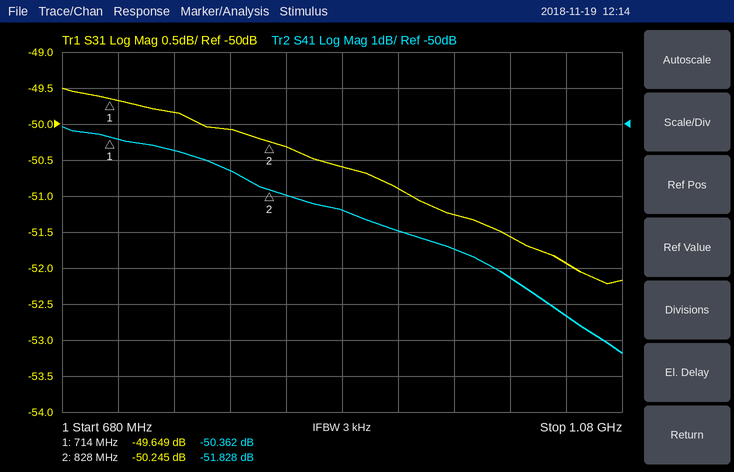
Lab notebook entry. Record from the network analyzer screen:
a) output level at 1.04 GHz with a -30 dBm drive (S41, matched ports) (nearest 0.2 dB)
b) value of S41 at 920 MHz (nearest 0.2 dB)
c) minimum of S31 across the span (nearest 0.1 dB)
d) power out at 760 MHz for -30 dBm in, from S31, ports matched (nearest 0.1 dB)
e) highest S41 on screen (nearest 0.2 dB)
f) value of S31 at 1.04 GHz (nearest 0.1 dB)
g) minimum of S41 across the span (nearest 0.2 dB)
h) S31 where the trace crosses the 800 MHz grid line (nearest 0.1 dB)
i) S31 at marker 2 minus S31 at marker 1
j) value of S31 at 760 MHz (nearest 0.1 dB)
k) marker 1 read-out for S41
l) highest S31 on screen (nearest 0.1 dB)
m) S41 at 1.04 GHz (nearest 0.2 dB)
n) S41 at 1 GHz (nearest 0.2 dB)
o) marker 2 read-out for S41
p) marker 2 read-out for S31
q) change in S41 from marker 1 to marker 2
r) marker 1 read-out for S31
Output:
-85.4 dBm
-53.0 dB
-52.2 dB
-79.8 dBm
-50.0 dB
-51.9 dB
-56.4 dB
-50.1 dB
-0.596 dB
-49.8 dB
-50.362 dB
-49.5 dB
-55.4 dB
-54.2 dB
-51.828 dB
-50.245 dB
-1.466 dB
-49.649 dB
